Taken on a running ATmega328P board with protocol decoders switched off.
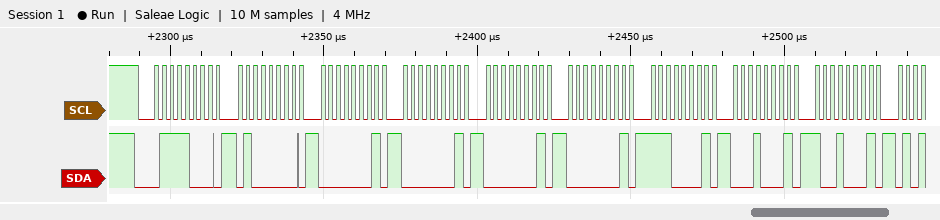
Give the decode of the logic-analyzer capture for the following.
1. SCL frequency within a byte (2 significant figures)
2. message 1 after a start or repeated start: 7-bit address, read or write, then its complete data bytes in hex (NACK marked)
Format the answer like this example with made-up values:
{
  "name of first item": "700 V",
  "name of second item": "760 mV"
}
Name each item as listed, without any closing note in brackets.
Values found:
{
  "SCL frequency within a byte": "400 kHz",
  "message 1 after a start or repeated start: 7-bit address, read or write, then its complete data bytes in hex": "0x3C write: 40 01 01 01 01 E1 11 91"
}
